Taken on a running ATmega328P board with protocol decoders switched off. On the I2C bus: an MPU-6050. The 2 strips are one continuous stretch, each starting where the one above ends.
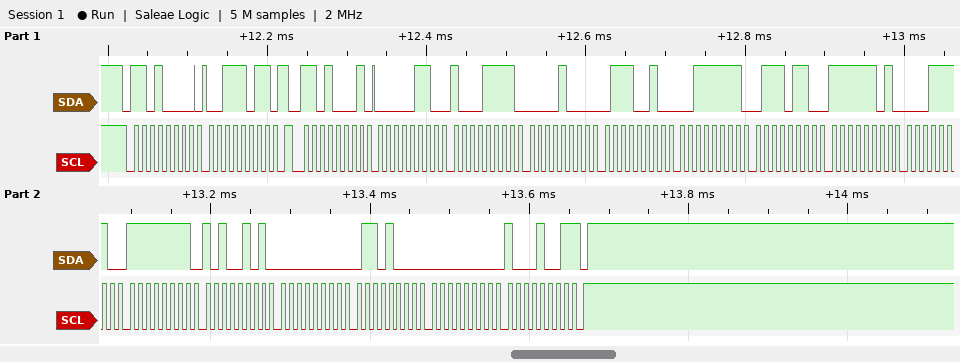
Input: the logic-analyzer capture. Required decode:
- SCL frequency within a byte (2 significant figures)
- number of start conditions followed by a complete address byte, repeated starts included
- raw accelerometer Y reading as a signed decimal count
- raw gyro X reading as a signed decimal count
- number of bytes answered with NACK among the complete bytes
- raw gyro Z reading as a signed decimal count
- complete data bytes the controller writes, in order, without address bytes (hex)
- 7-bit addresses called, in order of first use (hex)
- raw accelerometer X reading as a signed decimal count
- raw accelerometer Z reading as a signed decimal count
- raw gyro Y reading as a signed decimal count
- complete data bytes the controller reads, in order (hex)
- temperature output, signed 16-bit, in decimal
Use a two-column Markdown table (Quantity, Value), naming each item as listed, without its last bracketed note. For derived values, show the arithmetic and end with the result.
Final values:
| Quantity | Value |
|---|---|
| SCL frequency within a byte | 100 kHz |
| number of start conditions followed by a complete address byte, repeated starts included | 2 |
| raw accelerometer Y reading as a signed decimal count | 0x0872 = 2162 |
| raw gyro X reading as a signed decimal count | 0xFFA5 = -91 |
| number of bytes answered with NACK among the complete bytes | 1 |
| raw gyro Z reading as a signed decimal count | 0x0089 = 137 |
| complete data bytes the controller writes, in order, without address bytes | 3B |
| 7-bit addresses called, in order of first use | 0x68 |
| raw accelerometer X reading as a signed decimal count | 0x068F = 1679 |
| raw accelerometer Z reading as a signed decimal count | 0x3F76 = 16246 |
| raw gyro Y reading as a signed decimal count | 0x0068 = 104 |
| complete data bytes the controller reads, in order | 06 8F 08 72 3F 76 FD 1E FF A5 00 68 00 89 |
| temperature output, signed 16-bit, in decimal | 0xFD1E = -738 |
